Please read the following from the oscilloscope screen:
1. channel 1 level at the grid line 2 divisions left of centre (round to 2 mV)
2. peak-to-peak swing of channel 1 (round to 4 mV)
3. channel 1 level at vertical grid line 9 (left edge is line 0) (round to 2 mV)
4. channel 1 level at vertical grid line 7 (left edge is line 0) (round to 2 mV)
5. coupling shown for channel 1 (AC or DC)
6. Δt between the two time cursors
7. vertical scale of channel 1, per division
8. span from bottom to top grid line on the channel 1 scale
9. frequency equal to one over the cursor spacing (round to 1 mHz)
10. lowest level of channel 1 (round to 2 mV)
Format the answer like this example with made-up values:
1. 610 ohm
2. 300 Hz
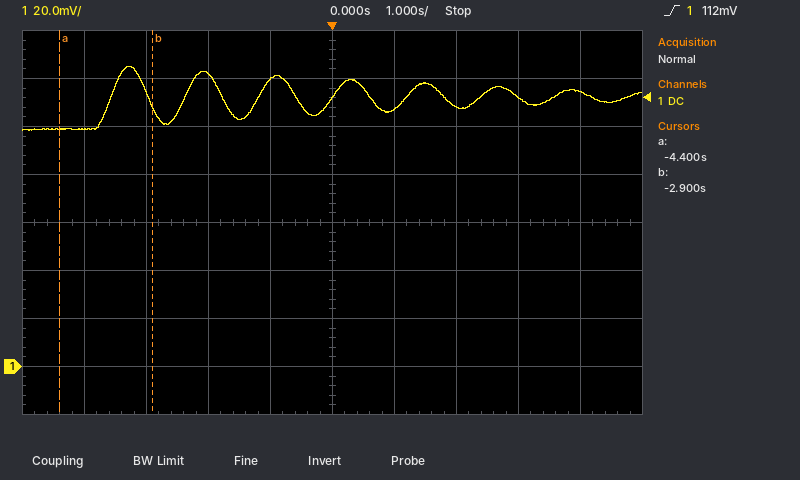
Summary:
1. 122 mV
2. 28 mV
3. 114 mV
4. 108 mV
5. DC
6. 1.5 s
7. 20 mV
8. 160 mV
9. 667 mHz
10. 98 mV
